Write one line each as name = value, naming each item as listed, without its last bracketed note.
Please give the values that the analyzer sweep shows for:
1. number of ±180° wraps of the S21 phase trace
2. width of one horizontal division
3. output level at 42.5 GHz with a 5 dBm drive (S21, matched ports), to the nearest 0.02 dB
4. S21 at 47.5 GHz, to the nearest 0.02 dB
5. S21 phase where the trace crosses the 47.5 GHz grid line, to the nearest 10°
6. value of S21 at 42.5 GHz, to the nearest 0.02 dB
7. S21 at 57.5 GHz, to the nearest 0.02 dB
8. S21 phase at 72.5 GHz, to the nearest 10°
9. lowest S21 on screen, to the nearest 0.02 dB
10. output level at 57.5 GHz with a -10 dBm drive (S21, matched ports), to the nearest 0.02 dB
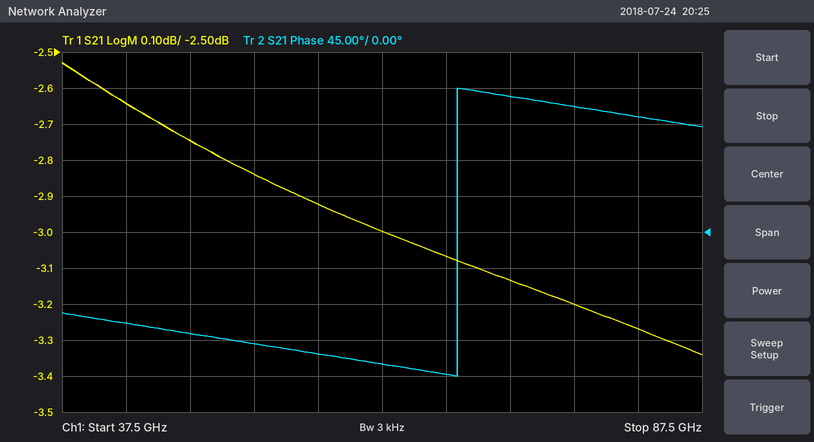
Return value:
number of ±180° wraps of the S21 phase trace = 1
width of one horizontal division = 5 GHz
output level at 42.5 GHz with a 5 dBm drive (S21, matched ports), to the nearest 0.02 dB = 2.36 dBm
S21 at 47.5 GHz, to the nearest 0.02 dB = -2.74 dB
S21 phase where the trace crosses the 47.5 GHz grid line, to the nearest 10° = -130°
value of S21 at 42.5 GHz, to the nearest 0.02 dB = -2.64 dB
S21 at 57.5 GHz, to the nearest 0.02 dB = -2.92 dB
S21 phase at 72.5 GHz, to the nearest 10° = 170°
lowest S21 on screen, to the nearest 0.02 dB = -3.34 dB
output level at 57.5 GHz with a -10 dBm drive (S21, matched ports), to the nearest 0.02 dB = -12.92 dBm
